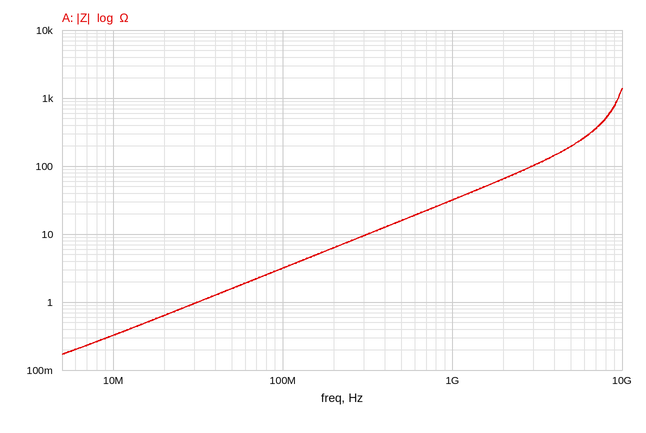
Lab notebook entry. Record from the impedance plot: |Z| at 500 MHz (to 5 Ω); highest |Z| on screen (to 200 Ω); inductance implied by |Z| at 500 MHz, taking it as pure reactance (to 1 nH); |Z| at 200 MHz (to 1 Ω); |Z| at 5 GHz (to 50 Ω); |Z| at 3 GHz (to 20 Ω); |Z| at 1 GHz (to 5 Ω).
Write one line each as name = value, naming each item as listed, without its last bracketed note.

|Z| at 500 MHz = 15 Ω
highest |Z| on screen = 1.4 kΩ
inductance implied by |Z| at 500 MHz, taking it as pure reactance = 5 nH
|Z| at 200 MHz = 6 Ω
|Z| at 5 GHz = 200 Ω
|Z| at 3 GHz = 100 Ω
|Z| at 1 GHz = 30 Ω
